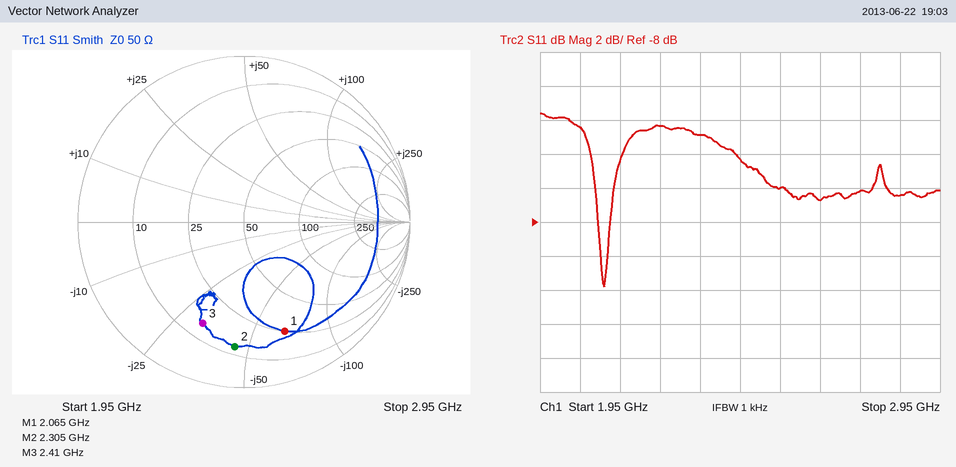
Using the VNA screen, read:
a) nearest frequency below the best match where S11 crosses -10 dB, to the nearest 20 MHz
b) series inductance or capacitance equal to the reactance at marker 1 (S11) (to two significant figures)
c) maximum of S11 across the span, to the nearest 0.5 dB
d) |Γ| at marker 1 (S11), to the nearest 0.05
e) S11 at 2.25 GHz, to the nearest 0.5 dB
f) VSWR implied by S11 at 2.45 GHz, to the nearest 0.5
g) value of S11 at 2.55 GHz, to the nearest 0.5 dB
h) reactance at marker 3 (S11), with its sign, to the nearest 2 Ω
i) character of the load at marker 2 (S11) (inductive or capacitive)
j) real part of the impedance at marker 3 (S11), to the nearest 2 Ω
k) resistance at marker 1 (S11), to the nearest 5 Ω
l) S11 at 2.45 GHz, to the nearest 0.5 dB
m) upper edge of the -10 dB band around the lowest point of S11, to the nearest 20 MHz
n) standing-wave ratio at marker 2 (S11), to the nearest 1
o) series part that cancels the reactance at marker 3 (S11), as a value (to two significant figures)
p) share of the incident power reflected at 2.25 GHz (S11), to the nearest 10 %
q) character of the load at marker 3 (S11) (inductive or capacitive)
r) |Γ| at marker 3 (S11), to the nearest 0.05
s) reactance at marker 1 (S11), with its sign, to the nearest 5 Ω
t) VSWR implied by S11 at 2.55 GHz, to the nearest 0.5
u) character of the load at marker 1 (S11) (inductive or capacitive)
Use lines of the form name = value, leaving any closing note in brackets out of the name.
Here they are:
nearest frequency below the best match where S11 crosses -10 dB, to the nearest 20 MHz = 2.10 GHz
series inductance or capacitance equal to the reactance at marker 1 (S11) = 1.2 pF
maximum of S11 across the span, to the nearest 0.5 dB = -1.5 dB
|Γ| at marker 1 (S11), to the nearest 0.05 = 0.70
S11 at 2.25 GHz, to the nearest 0.5 dB = -2.5 dB
VSWR implied by S11 at 2.45 GHz, to the nearest 0.5 = 4.0
value of S11 at 2.55 GHz, to the nearest 0.5 dB = -6.0 dB
reactance at marker 3 (S11), with its sign, to the nearest 2 Ω = -32 Ω
character of the load at marker 2 (S11) = capacitive
real part of the impedance at marker 3 (S11), to the nearest 2 Ω = 14 Ω
resistance at marker 1 (S11), to the nearest 5 Ω = 25 Ω
S11 at 2.45 GHz, to the nearest 0.5 dB = -4.5 dB
upper edge of the -10 dB band around the lowest point of S11, to the nearest 20 MHz = 2.12 GHz
standing-wave ratio at marker 2 (S11), to the nearest 1 = 7
series part that cancels the reactance at marker 3 (S11), as a value = 2.1 nH
share of the incident power reflected at 2.25 GHz (S11), to the nearest 10 % = 60 %
character of the load at marker 3 (S11) = capacitive
|Γ| at marker 3 (S11), to the nearest 0.05 = 0.65
reactance at marker 1 (S11), with its sign, to the nearest 5 Ω = -65 Ω
VSWR implied by S11 at 2.55 GHz, to the nearest 0.5 = 3.0
character of the load at marker 1 (S11) = capacitive
